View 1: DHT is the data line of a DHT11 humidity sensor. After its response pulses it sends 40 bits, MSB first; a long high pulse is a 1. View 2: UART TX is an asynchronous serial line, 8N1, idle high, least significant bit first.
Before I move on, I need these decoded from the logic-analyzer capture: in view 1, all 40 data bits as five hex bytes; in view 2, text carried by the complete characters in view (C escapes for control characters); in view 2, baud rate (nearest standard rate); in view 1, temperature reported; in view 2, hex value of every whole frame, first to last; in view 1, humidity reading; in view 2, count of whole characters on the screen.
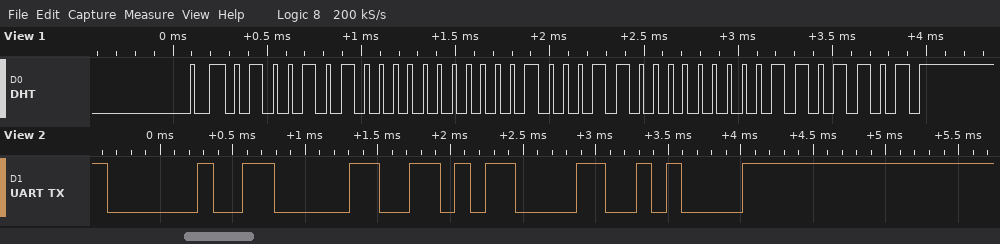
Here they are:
4A 00 23 00 6D
" 0\r\n"
9600 baud
35.0 °C
20 30 0D 0A
74 %
4
